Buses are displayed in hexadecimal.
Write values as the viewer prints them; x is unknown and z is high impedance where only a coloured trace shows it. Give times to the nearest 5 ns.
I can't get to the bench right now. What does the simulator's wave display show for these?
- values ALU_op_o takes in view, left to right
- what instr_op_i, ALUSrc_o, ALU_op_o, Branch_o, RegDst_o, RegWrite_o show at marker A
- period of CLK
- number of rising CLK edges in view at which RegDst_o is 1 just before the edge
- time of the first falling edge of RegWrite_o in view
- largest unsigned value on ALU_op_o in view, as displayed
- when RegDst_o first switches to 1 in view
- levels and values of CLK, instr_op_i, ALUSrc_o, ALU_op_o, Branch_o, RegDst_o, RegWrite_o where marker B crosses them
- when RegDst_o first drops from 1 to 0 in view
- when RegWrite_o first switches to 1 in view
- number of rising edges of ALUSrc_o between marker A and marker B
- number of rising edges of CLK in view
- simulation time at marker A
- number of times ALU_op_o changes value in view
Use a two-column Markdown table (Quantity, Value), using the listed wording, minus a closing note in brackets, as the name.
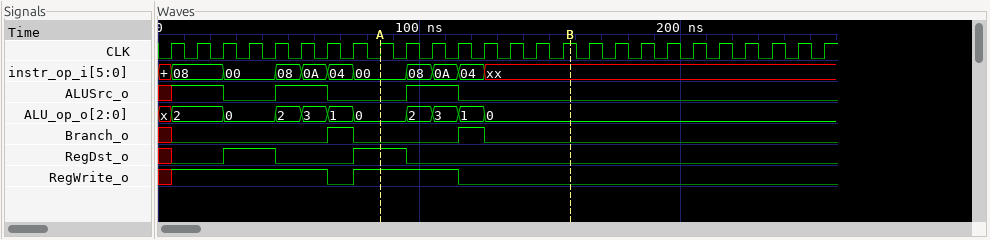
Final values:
| Quantity | Value |
|---|---|
| values ALU_op_o takes in view, left to right | x, 2, 0, 2, 3, 1, 0, 2, 3, 1, 0 |
| what instr_op_i, ALUSrc_o, ALU_op_o, Branch_o, RegDst_o, RegWrite_o show at marker A | instr_op_i=00, ALUSrc_o=0, ALU_op_o=0, Branch_o=0, RegDst_o=1, RegWrite_o=1 |
| period of CLK | 10 ns |
| number of rising CLK edges in view at which RegDst_o is 1 just before the edge | 4 |
| time of the first falling edge of RegWrite_o in view | 65 ns |
| largest unsigned value on ALU_op_o in view, as displayed | 3 |
| when RegDst_o first switches to 1 in view | 25 ns |
| levels and values of CLK, instr_op_i, ALUSrc_o, ALU_op_o, Branch_o, RegDst_o, RegWrite_o where marker B crosses them | CLK=1, instr_op_i=xx, ALUSrc_o=0, ALU_op_o=0, Branch_o=0, RegDst_o=0, RegWrite_o=0 |
| when RegDst_o first drops from 1 to 0 in view | 45 ns |
| when RegWrite_o first switches to 1 in view | 5 ns |
| number of rising edges of ALUSrc_o between marker A and marker B | 1 |
| number of rising edges of CLK in view | 26 |
| simulation time at marker A | 85 ns |
| number of times ALU_op_o changes value in view | 10 |
